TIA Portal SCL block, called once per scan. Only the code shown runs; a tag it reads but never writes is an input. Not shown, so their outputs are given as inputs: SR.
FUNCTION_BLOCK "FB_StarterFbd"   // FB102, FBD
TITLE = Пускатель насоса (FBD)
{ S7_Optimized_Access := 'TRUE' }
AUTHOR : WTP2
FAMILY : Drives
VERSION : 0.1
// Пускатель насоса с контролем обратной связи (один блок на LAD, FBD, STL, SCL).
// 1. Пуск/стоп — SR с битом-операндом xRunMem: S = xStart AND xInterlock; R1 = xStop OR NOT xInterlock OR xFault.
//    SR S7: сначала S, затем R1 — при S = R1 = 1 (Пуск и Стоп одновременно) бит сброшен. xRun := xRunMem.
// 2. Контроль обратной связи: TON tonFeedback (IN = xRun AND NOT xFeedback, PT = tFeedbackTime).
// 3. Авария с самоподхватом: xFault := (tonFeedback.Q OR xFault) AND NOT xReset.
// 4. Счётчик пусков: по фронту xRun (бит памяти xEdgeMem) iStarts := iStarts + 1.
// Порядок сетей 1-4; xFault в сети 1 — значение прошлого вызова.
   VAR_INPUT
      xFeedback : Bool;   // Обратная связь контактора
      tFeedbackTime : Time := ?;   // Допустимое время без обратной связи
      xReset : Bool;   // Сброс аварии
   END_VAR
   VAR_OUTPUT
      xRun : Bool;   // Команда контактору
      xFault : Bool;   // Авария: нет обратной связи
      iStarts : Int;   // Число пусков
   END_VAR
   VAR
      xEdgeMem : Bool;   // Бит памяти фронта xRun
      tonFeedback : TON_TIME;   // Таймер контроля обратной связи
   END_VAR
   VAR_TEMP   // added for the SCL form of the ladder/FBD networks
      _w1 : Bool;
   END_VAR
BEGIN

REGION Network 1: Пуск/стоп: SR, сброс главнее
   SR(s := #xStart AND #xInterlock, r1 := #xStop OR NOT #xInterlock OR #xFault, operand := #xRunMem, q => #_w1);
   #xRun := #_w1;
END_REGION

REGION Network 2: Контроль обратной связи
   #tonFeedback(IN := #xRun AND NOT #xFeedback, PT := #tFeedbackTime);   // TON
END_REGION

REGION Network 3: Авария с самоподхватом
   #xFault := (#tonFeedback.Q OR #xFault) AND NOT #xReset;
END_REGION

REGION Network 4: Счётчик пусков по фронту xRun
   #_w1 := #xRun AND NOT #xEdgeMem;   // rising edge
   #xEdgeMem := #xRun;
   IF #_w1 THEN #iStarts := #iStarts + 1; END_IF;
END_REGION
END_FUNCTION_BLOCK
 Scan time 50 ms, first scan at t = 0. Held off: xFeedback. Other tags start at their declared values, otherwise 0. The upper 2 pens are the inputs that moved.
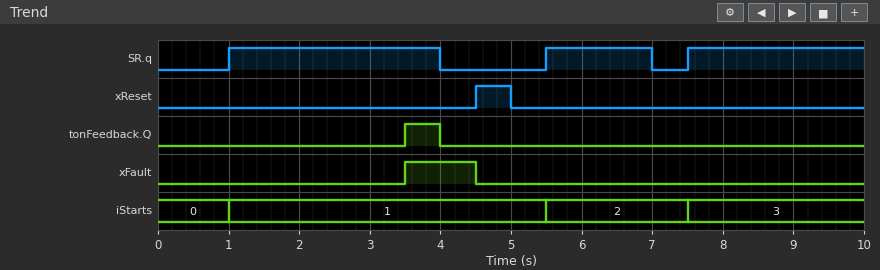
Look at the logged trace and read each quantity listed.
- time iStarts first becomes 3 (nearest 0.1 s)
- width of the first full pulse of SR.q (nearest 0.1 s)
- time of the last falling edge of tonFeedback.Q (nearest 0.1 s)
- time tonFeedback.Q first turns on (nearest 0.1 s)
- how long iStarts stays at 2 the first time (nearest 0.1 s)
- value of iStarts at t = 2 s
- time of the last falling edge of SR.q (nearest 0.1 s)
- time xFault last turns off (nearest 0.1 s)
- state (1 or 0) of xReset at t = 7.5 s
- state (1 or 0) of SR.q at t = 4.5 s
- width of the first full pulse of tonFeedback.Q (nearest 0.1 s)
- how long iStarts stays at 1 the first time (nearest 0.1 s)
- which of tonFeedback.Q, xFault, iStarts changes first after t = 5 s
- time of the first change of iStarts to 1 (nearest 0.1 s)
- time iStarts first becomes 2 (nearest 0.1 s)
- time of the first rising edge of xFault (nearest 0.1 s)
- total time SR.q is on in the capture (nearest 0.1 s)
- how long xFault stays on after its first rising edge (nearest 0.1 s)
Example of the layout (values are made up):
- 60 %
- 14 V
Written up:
- 7.5 s
- 3.0 s
- 4.0 s
- 3.5 s
- 2.0 s
- 1
- 7.0 s
- 4.5 s
- 0
- 0
- 0.5 s
- 4.5 s
- iStarts
- 1.0 s
- 5.5 s
- 3.5 s
- 7.0 s
- 1.0 s
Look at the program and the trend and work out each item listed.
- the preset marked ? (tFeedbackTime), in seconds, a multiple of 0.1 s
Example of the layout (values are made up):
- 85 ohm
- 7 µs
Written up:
- 2.5 s
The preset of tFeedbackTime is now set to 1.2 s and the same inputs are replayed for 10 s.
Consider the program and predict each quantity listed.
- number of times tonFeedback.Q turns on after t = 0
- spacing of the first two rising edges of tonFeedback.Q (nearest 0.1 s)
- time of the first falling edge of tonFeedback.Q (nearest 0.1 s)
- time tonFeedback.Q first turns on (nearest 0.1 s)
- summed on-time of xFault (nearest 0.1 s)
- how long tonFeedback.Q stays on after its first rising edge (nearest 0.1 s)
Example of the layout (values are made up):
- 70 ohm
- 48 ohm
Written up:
- 3
- 4.5 s
- 4.0 s
- 2.2 s
- 5.6 s
- 1.8 s
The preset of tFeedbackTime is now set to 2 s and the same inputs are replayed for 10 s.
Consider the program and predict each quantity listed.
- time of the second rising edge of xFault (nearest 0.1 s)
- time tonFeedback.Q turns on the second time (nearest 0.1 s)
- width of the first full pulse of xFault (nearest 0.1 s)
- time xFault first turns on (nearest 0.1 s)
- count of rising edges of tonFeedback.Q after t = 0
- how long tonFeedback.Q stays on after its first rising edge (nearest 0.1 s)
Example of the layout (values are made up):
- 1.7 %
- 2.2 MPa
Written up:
- 9.5 s
- 9.5 s
- 1.5 s
- 3.0 s
- 2
- 1.0 s
